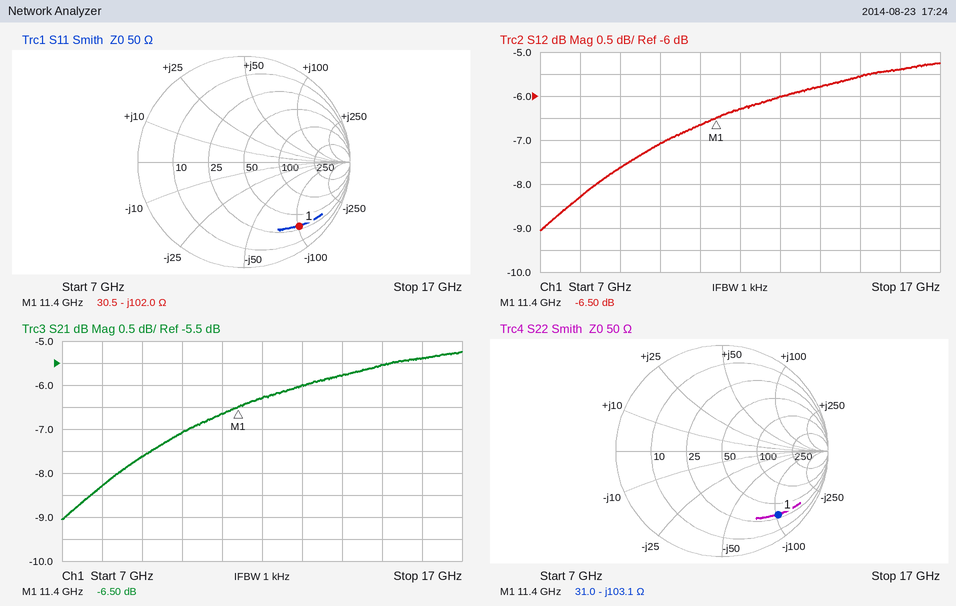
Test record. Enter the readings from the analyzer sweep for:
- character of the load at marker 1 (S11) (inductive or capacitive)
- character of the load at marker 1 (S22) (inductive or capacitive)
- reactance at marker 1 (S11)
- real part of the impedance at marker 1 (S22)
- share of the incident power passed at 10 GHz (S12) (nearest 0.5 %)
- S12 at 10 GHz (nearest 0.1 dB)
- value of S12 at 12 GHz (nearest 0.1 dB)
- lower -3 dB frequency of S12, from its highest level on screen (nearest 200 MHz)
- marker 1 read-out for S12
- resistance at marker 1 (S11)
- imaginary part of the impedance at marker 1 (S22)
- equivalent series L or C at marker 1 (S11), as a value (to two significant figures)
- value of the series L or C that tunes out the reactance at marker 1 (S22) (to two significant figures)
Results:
capacitive
capacitive
-102.0 Ω
31.0 Ω
19.5 %
-7.1 dB
-6.3 dB
8.0 GHz
-6.50 dB
30.5 Ω
-103.1 Ω
140 fF
1.4 nH
